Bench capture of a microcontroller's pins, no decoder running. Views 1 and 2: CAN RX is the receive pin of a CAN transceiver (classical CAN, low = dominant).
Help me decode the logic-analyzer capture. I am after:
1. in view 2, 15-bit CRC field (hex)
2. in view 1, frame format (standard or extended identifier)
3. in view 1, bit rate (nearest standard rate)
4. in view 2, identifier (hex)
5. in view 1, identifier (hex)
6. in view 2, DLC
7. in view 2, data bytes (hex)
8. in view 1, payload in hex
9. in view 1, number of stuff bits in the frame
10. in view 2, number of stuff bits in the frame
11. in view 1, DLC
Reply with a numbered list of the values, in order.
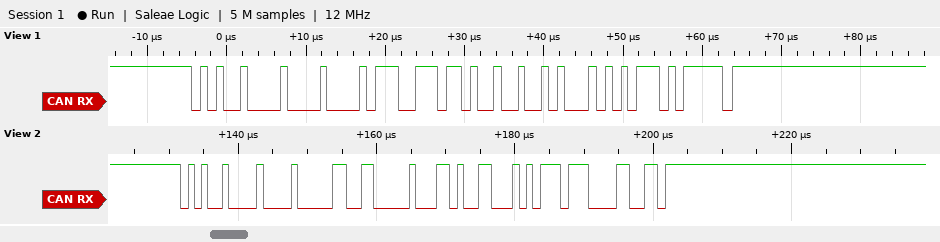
1. 0x6E19
2. standard
3. 1000 kbit/s
4. 0x521
5. 0x521
6. 4
7. 13 00 D3 15
8. 2E 76 92 51
9. 0
10. 2
11. 4
